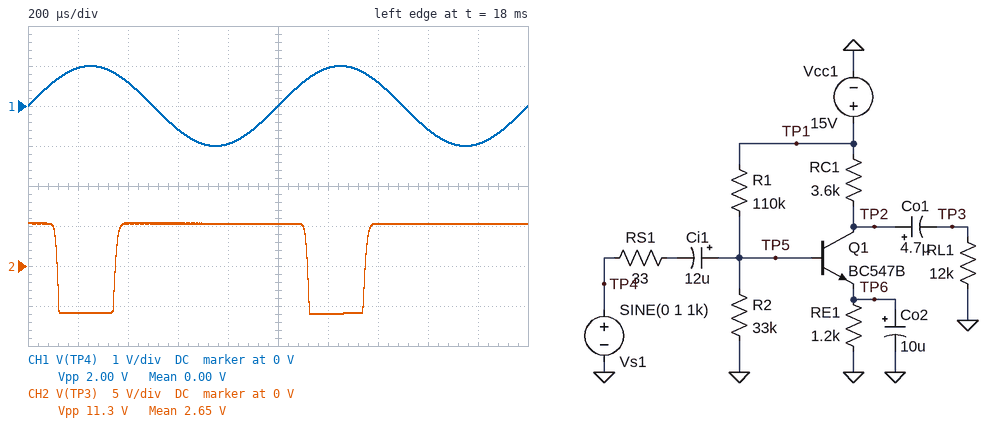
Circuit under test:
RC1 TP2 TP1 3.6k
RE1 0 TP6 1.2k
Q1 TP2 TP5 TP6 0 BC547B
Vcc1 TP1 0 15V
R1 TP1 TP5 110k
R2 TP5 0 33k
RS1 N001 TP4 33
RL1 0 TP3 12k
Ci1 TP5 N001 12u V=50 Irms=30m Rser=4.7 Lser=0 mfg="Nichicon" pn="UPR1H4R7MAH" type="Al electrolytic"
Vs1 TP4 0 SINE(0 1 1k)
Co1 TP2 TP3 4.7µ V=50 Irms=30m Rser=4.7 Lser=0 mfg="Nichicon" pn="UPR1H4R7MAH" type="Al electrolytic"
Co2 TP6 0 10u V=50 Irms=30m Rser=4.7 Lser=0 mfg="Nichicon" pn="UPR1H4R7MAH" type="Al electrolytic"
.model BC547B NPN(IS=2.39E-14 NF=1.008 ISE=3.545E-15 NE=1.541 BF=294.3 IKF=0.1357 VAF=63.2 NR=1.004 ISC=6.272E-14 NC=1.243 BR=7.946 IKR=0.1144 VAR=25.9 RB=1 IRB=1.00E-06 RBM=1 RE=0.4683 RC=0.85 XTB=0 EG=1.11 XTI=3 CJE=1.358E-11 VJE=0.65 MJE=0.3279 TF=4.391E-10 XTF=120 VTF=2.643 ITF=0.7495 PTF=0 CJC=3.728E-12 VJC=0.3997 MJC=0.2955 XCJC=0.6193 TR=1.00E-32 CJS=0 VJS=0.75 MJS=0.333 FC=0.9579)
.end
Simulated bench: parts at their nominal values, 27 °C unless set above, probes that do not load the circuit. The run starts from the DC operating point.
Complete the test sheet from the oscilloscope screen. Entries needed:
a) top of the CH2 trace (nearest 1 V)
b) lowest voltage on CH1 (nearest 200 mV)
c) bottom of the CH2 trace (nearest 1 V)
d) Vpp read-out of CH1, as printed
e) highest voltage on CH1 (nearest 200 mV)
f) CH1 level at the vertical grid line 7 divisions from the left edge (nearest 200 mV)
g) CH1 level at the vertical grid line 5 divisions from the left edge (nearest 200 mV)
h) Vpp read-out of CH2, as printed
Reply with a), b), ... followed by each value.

a) 5 V
b) -1.0 V
c) -6 V
d) 2.00 V
e) 1.0 V
f) 600 mV
g) 0 V
h) 11.3 V
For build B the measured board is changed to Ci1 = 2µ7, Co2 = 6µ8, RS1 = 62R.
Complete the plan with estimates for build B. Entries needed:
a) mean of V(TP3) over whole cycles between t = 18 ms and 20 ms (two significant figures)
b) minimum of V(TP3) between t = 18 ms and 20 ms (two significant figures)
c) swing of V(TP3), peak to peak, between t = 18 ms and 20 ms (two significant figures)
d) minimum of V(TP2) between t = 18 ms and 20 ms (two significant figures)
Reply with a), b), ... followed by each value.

a) 2.9 V
b) -6.7 V
c) 12 V
d) 1.5 V
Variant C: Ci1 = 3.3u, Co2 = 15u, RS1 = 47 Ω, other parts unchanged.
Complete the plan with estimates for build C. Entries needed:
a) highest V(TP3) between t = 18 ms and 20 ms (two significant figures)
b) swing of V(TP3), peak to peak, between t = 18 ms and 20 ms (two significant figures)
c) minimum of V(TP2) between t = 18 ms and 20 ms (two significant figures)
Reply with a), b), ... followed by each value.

a) 5.2 V
b) 12 V
c) 1.8 V
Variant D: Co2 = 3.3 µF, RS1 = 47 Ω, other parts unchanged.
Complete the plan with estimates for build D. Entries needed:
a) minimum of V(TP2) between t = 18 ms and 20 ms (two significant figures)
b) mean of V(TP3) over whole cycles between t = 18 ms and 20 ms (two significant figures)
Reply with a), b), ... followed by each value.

a) 1.9 V
b) 2.4 V
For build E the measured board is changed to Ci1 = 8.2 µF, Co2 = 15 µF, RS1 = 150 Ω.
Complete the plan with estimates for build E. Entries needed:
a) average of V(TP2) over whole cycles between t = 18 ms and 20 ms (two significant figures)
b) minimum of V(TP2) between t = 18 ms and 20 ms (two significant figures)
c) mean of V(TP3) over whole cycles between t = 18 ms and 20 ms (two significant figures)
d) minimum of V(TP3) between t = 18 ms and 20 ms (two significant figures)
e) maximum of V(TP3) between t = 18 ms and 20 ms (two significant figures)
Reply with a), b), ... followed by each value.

a) 10 V
b) 2.2 V
c) 2.3 V
d) -5.7 V
e) 5.5 V
